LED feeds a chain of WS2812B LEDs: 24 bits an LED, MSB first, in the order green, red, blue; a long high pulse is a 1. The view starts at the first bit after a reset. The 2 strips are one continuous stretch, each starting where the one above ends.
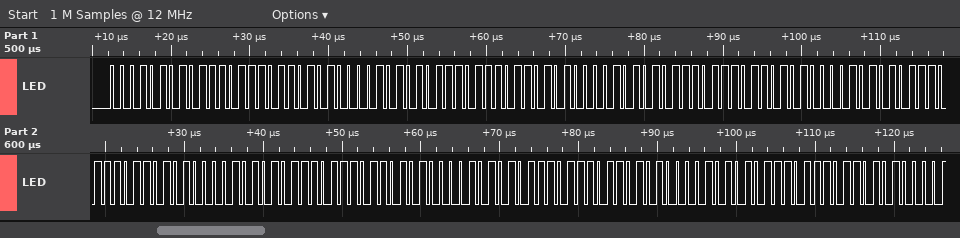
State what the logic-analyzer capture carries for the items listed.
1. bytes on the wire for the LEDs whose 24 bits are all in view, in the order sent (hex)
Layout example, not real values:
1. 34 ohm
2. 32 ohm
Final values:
1. 15 77 6A 15 77 6A 15 77 6A 15 77 6A 15 77 6A 15 77 6A 15 77 6A
